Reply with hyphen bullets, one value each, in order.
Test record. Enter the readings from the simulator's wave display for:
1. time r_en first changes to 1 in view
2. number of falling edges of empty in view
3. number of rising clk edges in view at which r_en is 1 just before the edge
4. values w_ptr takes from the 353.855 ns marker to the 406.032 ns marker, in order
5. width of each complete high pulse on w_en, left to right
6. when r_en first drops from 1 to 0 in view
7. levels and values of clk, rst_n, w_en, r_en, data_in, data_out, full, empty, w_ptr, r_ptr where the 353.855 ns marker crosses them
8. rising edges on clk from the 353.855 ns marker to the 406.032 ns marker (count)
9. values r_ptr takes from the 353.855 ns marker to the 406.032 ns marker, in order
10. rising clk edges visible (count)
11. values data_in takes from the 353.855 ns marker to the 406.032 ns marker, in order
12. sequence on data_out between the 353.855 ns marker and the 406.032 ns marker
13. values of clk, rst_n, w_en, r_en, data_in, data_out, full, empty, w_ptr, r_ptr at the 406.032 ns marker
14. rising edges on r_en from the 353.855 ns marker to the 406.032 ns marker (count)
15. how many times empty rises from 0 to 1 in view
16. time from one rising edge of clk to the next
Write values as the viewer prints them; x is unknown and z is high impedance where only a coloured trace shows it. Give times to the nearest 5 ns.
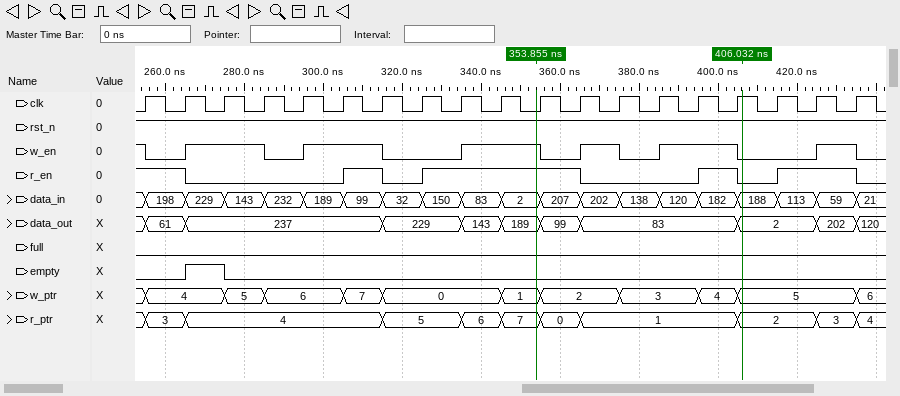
- 305 ns
- 1
- 10
- 1, 2, 3, 4, 5
- 20 ns, 20 ns, 20 ns, 10 ns, 20 ns, 10 ns
- 265 ns
- clk=0, rst_n=1, w_en=1, r_en=1, data_in=2, data_out=189, full=0, empty=0, w_ptr=1, r_ptr=7
- 6
- 7, 0, 1, 2
- 19
- 2, 207, 202, 138, 120, 182, 188
- 189, 99, 83, 2
- clk=1, rst_n=1, w_en=0, r_en=0, data_in=188, data_out=2, full=0, empty=0, w_ptr=5, r_ptr=2
- 1
- 1
- 10 ns
